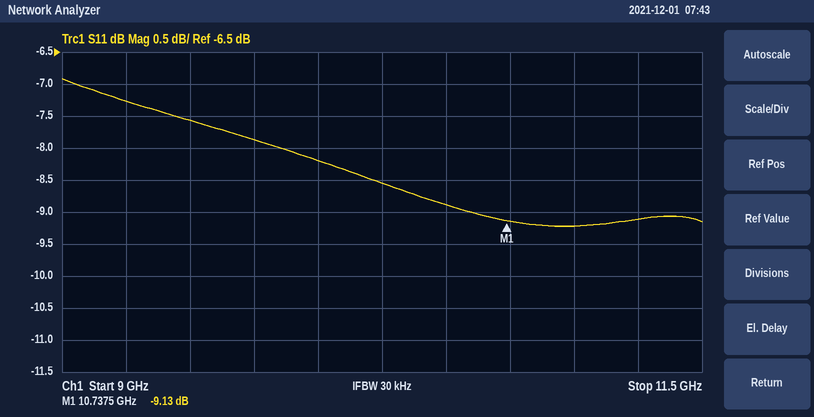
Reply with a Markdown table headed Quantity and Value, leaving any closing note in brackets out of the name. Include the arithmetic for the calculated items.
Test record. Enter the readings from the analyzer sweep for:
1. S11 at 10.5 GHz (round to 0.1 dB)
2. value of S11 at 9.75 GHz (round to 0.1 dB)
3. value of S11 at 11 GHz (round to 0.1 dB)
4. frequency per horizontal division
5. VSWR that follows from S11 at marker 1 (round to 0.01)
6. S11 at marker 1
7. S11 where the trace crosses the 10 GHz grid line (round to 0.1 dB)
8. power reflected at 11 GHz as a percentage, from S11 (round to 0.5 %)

| Quantity | Value |
|---|---|
| S11 at 10.5 GHz | -8.9 dB |
| value of S11 at 9.75 GHz | -7.9 dB |
| value of S11 at 11 GHz | -9.2 dB |
| frequency per horizontal division | 250 MHz |
| VSWR that follows from S11 at marker 1 | (1 + 0.3495)/(1 − 0.3495) ≈ 2.07 |
| S11 at marker 1 | -9.13 dB |
| S11 where the trace crosses the 10 GHz grid line | -8.2 dB |
| power reflected at 11 GHz as a percentage, from S11 | 10^(-9.2/10) ≈ 12.0 % |
